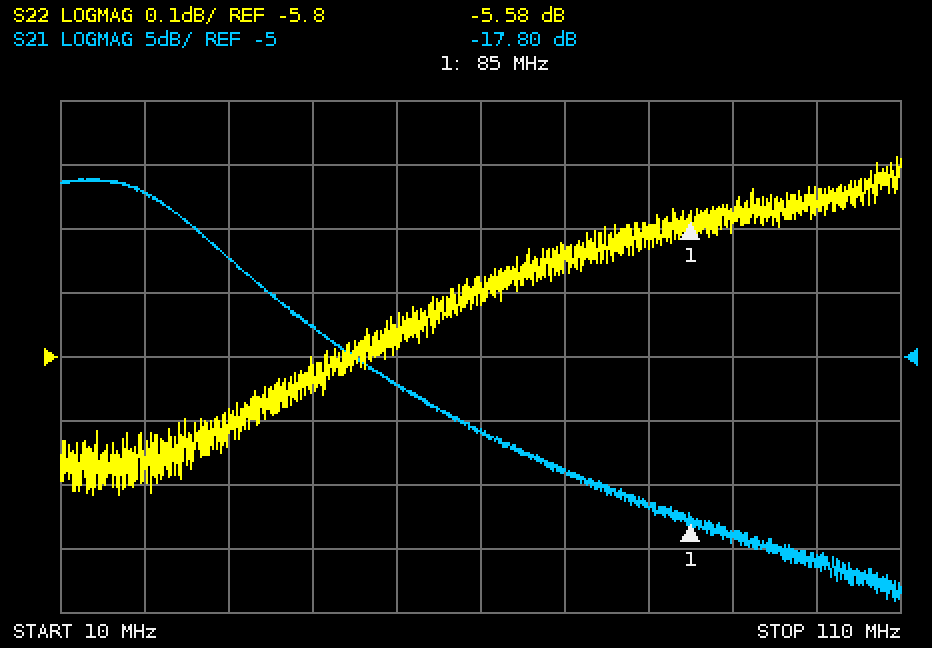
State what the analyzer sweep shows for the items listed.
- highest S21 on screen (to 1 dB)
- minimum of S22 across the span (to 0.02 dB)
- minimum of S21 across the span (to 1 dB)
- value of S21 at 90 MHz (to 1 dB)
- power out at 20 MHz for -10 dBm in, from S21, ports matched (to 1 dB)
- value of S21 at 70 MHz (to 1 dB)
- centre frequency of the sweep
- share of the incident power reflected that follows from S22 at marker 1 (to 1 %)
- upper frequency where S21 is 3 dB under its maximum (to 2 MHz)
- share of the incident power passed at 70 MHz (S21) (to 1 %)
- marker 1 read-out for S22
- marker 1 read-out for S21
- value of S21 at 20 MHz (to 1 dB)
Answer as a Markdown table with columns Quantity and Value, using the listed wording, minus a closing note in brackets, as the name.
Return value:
| Quantity | Value |
|---|---|
| highest S21 on screen | 9 dB |
| minimum of S22 across the span | -6.02 dB |
| minimum of S21 across the span | -24 dB |
| value of S21 at 90 MHz | -19 dB |
| power out at 20 MHz for -10 dBm in, from S21, ports matched | -2 dBm |
| value of S21 at 70 MHz | -14 dB |
| centre frequency of the sweep | 60 MHz |
| share of the incident power reflected that follows from S22 at marker 1 | 28 % |
| upper frequency where S21 is 3 dB under its maximum | 24 MHz |
| share of the incident power passed at 70 MHz (S21) | 4 % |
| marker 1 read-out for S22 | -5.58 dB |
| marker 1 read-out for S21 | -17.80 dB |
| value of S21 at 20 MHz | 8 dB |
